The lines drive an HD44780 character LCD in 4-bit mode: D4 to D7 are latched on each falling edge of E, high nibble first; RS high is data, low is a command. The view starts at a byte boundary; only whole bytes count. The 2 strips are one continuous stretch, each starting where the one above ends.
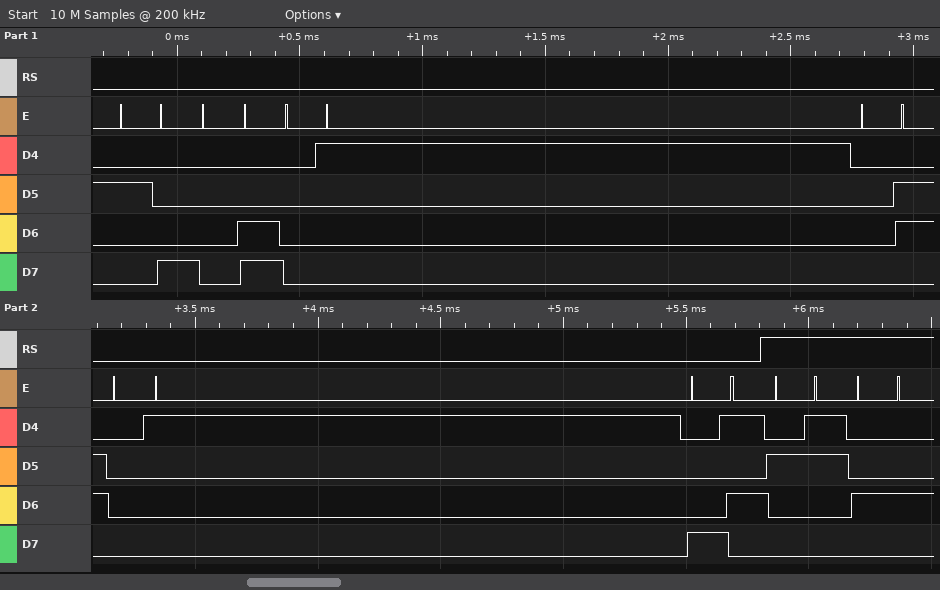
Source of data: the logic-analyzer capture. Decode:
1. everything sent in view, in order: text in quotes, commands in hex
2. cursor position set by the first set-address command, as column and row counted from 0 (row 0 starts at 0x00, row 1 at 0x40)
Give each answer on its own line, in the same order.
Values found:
0x28 0x0C 0x01 0x06 0x01 0x85 "#D"
column 5, row 0
